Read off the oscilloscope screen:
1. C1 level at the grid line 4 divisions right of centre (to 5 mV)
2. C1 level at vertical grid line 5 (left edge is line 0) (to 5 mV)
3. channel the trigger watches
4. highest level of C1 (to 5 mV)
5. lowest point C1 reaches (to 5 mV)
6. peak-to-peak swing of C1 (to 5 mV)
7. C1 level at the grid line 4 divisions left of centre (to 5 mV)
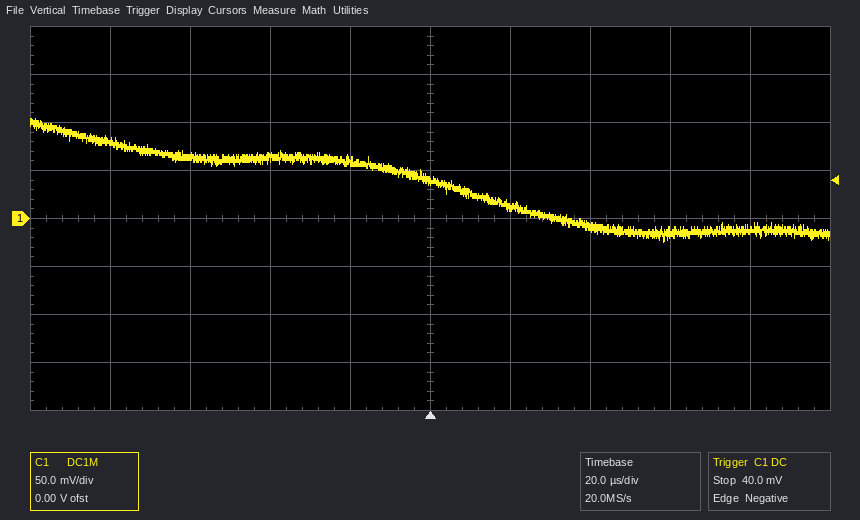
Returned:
-10 mV
40 mV
C1
105 mV
-25 mV
130 mV
80 mV
